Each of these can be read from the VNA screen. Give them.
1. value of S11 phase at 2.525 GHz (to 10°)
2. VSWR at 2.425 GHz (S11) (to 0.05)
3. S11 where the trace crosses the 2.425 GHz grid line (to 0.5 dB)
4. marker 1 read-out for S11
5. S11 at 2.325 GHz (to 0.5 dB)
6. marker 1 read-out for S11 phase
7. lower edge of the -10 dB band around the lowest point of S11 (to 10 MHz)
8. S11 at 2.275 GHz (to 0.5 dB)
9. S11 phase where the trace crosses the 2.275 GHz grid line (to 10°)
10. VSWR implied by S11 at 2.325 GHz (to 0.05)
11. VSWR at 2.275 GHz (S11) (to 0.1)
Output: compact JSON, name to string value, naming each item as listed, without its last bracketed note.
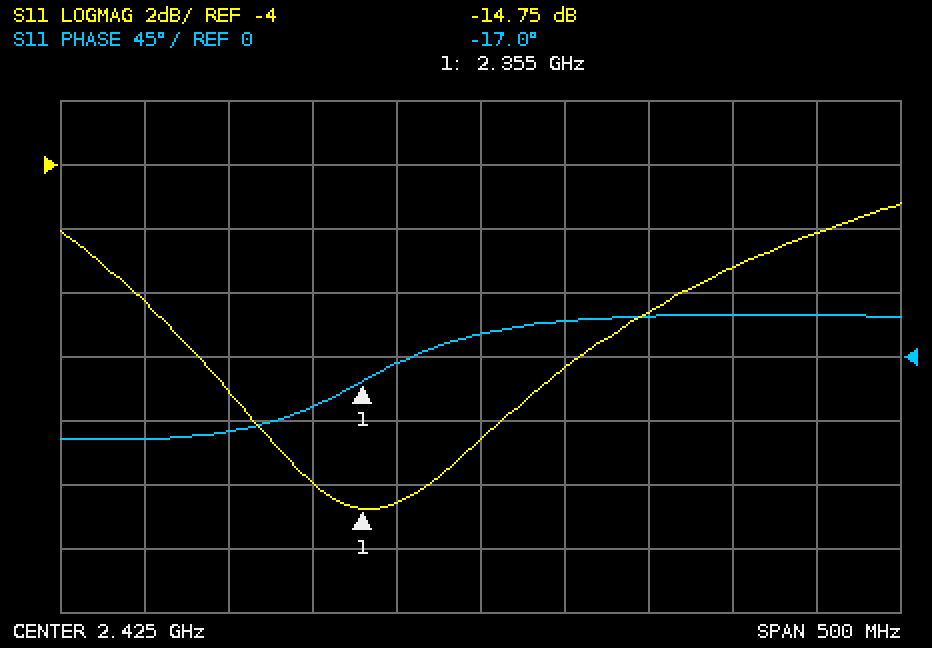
{"value of S11 phase at 2.525 GHz": "30°", "VSWR at 2.425 GHz (S11)": "1.60", "S11 where the trace crosses the 2.425 GHz grid line": "-12.5 dB", "marker 1 read-out for S11": "-14.75 dB", "S11 at 2.325 GHz": "-14.0 dB", "marker 1 read-out for S11 phase": "-17.0°", "lower edge of the -10 dB band around the lowest point of S11": "2.26 GHz", "S11 at 2.275 GHz": "-11.0 dB", "S11 phase where the trace crosses the 2.275 GHz grid line": "-50°", "VSWR implied by S11 at 2.325 GHz": "1.50", "VSWR at 2.275 GHz (S11)": "1.8"}
